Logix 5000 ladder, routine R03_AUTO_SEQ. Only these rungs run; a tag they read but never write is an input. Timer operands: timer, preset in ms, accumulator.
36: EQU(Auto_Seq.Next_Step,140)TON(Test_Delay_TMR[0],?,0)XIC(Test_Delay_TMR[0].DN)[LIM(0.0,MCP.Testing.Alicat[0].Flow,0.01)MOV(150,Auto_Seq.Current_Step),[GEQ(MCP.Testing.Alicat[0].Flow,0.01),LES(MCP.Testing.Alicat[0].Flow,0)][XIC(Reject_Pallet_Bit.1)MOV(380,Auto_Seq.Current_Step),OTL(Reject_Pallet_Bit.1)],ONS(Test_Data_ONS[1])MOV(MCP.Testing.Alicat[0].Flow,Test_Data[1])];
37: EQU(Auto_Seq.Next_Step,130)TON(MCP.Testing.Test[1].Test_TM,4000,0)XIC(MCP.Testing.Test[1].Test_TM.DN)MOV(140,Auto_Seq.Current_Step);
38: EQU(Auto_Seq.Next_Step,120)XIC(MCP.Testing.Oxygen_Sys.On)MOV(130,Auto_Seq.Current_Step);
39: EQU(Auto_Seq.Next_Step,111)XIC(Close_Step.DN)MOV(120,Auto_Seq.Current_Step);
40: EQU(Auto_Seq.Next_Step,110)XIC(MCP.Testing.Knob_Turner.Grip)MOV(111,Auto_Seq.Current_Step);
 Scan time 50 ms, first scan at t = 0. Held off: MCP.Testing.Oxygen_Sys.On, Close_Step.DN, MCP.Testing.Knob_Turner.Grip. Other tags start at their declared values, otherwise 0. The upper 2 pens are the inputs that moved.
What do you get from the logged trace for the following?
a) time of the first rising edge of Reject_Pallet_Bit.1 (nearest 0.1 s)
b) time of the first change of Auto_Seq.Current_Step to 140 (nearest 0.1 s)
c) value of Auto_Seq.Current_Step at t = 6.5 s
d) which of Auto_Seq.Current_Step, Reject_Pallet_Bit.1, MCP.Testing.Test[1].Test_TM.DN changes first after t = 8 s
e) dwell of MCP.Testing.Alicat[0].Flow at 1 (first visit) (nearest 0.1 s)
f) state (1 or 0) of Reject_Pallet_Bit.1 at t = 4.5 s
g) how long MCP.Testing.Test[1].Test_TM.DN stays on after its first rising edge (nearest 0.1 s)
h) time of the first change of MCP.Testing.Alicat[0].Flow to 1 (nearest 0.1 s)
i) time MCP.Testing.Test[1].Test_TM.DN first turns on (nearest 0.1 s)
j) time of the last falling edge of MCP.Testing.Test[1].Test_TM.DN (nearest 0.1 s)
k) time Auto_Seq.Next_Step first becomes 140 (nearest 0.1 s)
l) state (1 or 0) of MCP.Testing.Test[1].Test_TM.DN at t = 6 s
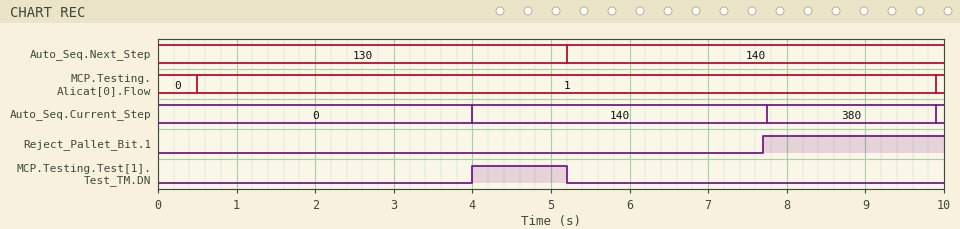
7.7 s
4.0 s
140
Auto_Seq.Current_Step
9.4 s
0
1.2 s
0.5 s
4.0 s
5.2 s
5.2 s
0
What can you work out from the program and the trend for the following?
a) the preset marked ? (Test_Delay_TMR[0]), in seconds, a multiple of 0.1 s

2.5 s
